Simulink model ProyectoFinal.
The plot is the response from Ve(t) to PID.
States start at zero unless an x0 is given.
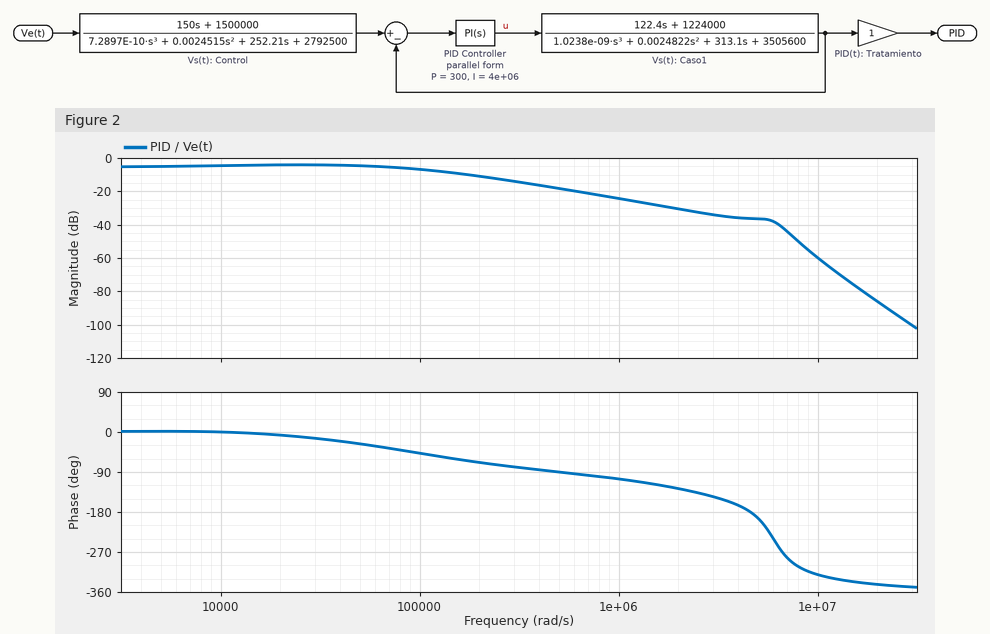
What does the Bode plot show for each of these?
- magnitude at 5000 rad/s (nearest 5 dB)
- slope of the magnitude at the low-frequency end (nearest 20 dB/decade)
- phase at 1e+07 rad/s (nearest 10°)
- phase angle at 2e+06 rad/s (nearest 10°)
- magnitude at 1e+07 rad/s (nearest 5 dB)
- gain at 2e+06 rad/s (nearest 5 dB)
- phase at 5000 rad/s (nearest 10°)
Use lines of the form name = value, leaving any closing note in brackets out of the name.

magnitude at 5000 rad/s = -5 dB
slope of the magnitude at the low-frequency end = 0 dB/decade
phase at 1e+07 rad/s = -320°
phase angle at 2e+06 rad/s = -130°
magnitude at 1e+07 rad/s = -60 dB
gain at 2e+06 rad/s = -30 dB
phase at 5000 rad/s = 0°
